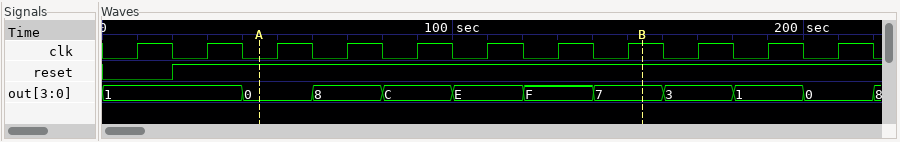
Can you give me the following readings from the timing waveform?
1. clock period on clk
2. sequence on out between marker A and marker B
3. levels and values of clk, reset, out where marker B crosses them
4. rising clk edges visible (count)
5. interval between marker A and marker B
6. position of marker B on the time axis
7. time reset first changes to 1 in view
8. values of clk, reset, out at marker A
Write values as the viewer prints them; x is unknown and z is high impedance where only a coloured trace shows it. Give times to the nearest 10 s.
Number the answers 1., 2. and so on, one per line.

1. 20 s
2. 0, 8, C, E, F, 7
3. clk=1, reset=1, out=7
4. 11
5. 110 s
6. 150 s
7. 20 s
8. clk=0, reset=1, out=0
